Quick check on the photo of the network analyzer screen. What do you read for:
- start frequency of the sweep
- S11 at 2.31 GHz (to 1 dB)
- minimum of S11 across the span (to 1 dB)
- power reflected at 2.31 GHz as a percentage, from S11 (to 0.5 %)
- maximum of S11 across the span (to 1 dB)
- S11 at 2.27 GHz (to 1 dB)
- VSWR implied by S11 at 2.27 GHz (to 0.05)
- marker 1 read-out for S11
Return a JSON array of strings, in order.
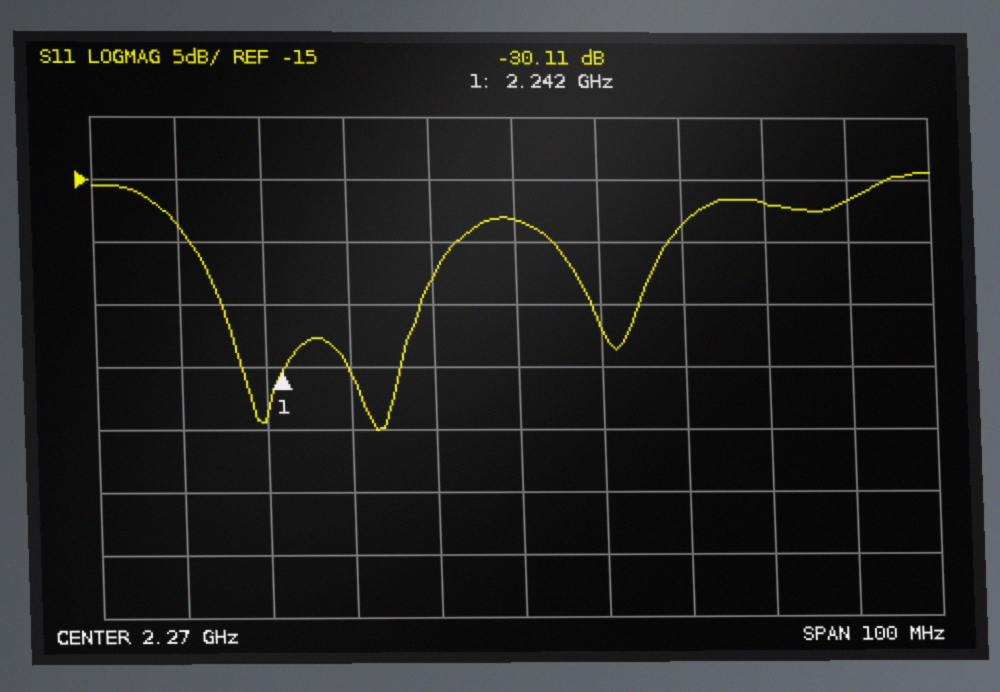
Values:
["2.22 GHz", "-17 dB", "-35 dB", "2.0 %", "-14 dB", "-18 dB", "1.30", "-30.11 dB"]
